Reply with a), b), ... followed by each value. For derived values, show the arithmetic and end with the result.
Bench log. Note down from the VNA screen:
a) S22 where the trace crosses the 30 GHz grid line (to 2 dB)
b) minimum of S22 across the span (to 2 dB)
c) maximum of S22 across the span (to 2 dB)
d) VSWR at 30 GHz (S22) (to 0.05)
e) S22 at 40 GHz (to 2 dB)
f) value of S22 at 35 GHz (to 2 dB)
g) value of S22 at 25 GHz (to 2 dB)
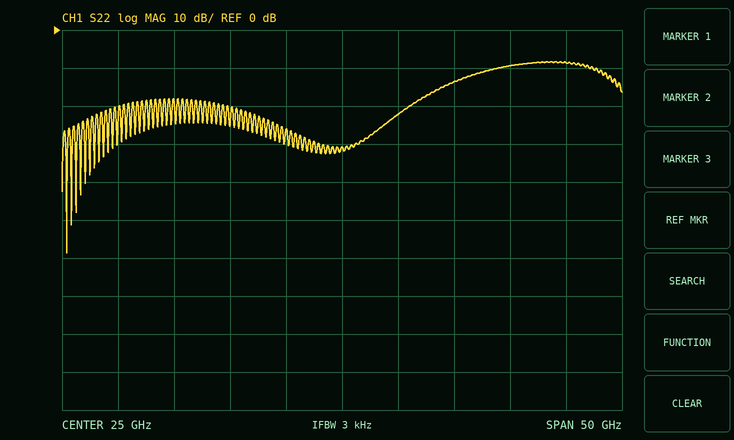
a) -22 dB
b) -58 dB
c) -8 dB
d) |Γ| = 10^(-22/20) = 0.0794; VSWR = (1 + 0.0794)/(1 − 0.0794) ≈ 1.17, so 1.15 to the nearest 0.05
e) -10 dB
f) -14 dB
g) -30 dB
